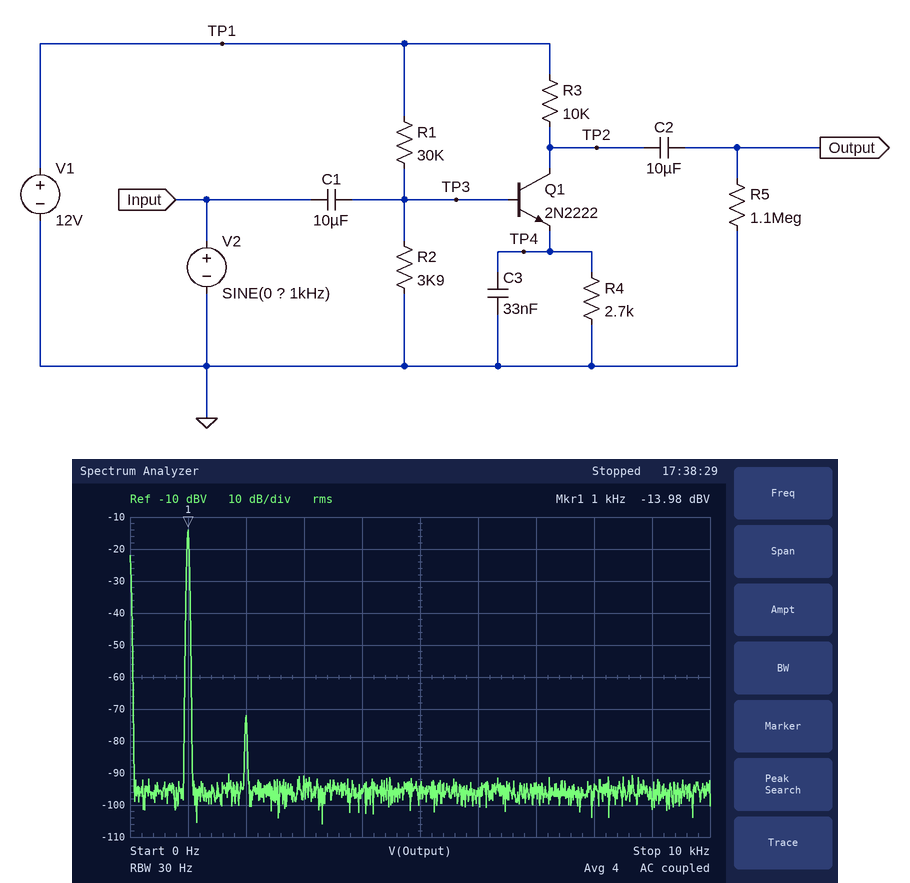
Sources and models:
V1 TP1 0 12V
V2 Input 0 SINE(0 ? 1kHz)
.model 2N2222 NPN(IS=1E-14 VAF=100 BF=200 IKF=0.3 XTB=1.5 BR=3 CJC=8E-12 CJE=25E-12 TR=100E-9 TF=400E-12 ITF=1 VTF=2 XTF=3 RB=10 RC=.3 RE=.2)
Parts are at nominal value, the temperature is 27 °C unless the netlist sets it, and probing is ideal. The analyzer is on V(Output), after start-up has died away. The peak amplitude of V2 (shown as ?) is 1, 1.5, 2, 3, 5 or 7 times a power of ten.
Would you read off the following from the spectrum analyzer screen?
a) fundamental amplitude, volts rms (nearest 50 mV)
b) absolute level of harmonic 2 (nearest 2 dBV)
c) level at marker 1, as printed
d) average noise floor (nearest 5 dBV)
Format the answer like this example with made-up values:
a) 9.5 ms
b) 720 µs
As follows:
a) 200 mV
b) -72 dBV
c) -13.98 dBV
d) -95 dBV
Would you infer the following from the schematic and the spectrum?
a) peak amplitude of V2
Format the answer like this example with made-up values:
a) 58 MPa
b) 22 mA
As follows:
a) 70 mV
